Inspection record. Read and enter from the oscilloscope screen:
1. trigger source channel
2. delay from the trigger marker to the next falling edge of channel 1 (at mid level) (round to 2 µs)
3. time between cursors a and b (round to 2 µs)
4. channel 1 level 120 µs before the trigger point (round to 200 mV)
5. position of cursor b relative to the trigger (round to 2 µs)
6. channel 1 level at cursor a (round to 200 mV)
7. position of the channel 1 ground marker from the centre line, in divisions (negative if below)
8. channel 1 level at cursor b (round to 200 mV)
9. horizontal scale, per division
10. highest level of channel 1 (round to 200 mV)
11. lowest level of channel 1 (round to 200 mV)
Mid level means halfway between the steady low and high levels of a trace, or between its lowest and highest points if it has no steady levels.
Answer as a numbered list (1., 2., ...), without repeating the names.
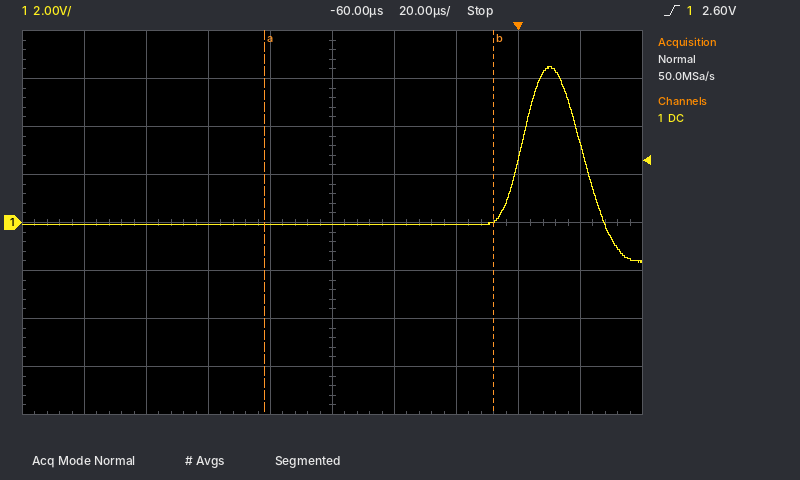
1. channel 1
2. 22 µs
3. 74 µs
4. 0.0 V
5. -8 µs
6. 0.0 V
7. 0.0 div
8. 0.0 V
9. 20 µs
10. 6.4 V
11. -1.6 V
